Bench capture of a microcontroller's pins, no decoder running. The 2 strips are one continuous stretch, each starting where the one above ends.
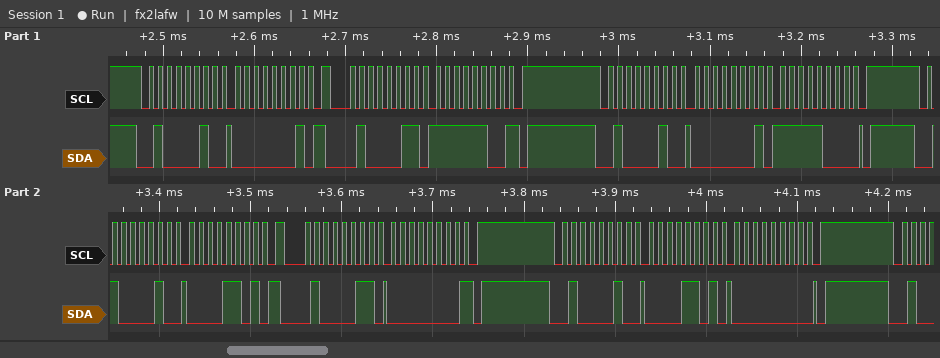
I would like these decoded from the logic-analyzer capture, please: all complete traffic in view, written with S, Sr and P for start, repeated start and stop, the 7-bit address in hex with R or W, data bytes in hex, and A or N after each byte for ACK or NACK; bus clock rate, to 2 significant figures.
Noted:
S 21W A 01 A Sr 21R A FC N P S 21W A 01 A F8 A P S 21W A 0D A Sr 21R A 00 N P S 21W A 0D A 00 A P
100 kHz
